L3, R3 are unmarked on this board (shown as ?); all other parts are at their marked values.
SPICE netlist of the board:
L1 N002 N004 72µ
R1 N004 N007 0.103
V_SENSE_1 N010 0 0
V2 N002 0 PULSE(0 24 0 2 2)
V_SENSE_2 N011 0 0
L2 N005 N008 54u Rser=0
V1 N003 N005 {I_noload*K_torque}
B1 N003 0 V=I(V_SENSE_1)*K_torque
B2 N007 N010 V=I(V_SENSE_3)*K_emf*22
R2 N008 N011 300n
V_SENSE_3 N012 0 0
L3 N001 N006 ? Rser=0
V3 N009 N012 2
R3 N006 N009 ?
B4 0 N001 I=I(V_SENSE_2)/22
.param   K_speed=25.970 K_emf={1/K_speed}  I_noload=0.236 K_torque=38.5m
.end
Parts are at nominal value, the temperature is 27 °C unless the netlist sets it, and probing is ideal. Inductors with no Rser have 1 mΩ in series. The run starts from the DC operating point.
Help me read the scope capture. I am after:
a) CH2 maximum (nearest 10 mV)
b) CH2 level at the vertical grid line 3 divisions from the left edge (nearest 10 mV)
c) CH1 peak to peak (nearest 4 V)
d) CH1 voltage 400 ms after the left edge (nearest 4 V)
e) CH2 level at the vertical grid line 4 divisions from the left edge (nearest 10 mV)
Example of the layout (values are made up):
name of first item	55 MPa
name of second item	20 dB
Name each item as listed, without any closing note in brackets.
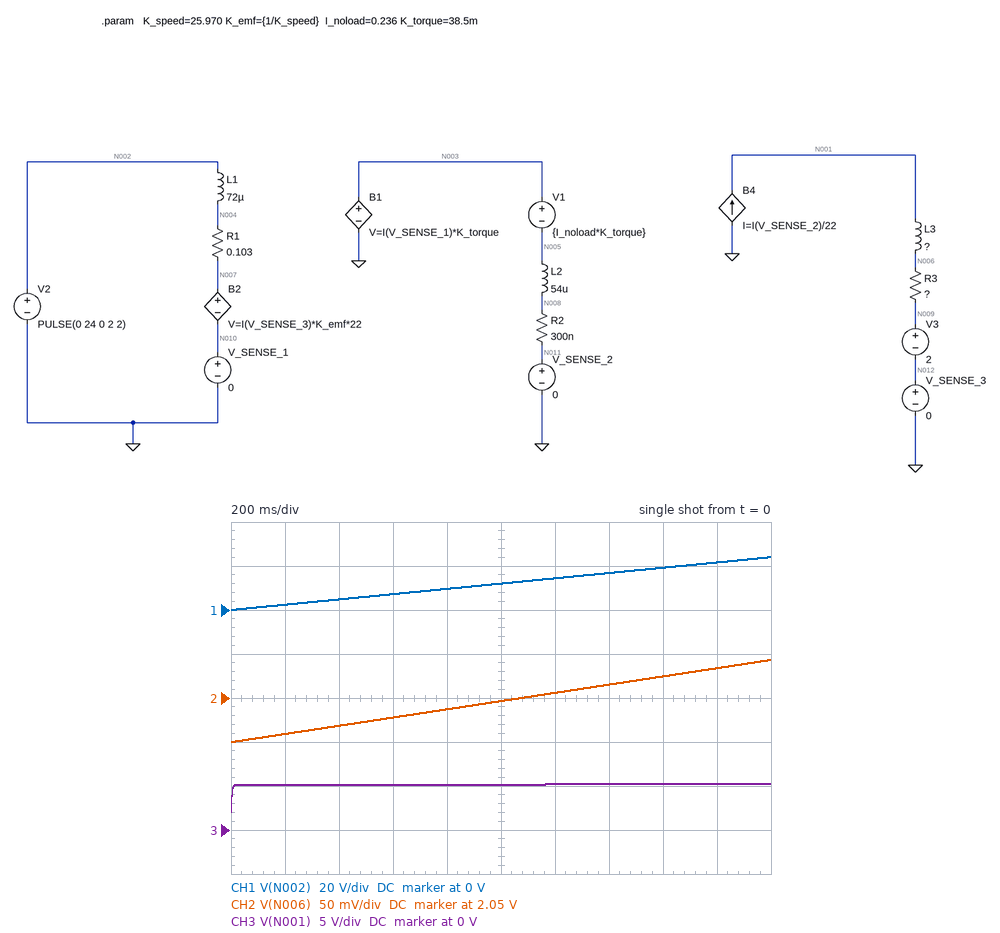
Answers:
CH2 maximum	2.09 V
CH2 level at the vertical grid line 3 divisions from the left edge	2.03 V
CH1 peak to peak	24 V
CH1 voltage 400 ms after the left edge	4 V
CH2 level at the vertical grid line 4 divisions from the left edge	2.04 V
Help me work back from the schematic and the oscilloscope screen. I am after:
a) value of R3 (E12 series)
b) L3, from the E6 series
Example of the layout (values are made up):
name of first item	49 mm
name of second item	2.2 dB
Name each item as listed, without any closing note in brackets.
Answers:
value of R3	3.3 mΩ
L3, from the E6 series	220 mH
